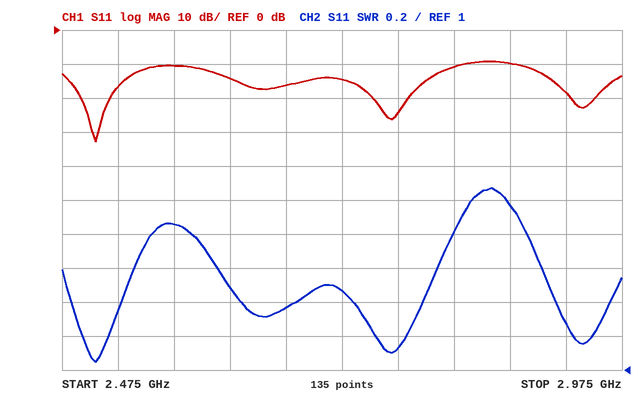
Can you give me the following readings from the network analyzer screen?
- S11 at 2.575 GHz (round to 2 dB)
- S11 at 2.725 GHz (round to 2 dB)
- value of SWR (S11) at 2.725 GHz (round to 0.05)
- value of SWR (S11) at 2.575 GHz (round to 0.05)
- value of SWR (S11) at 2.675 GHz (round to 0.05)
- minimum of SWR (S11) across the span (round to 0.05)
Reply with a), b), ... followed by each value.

a) -10 dB
b) -14 dB
c) 1.45
d) 1.85
e) 1.35
f) 1.05
